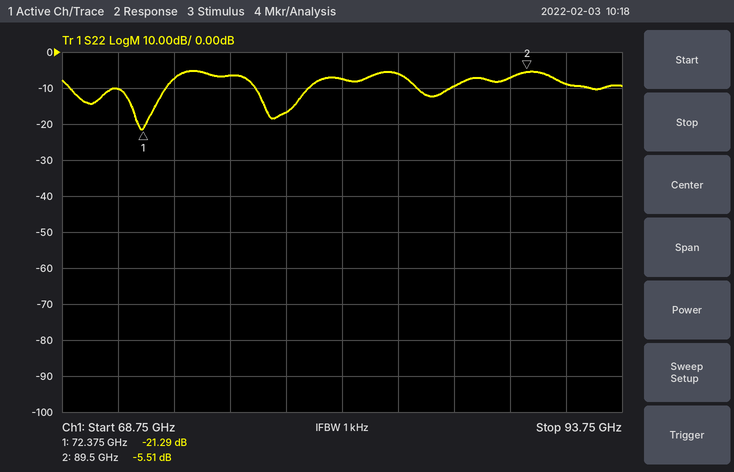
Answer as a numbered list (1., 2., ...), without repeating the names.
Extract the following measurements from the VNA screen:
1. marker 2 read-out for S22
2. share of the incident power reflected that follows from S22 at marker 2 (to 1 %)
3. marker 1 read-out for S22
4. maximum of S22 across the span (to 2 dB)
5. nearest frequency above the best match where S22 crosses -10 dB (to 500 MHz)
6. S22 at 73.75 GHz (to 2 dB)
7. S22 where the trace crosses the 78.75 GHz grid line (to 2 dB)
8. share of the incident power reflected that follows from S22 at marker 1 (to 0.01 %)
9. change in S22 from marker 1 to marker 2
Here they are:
1. -5.51 dB
2. 28 %
3. -21.29 dB
4. -6 dB
5. 73.5 GHz
6. -8 dB
7. -16 dB
8. 0.74 %
9. 15.78 dB
